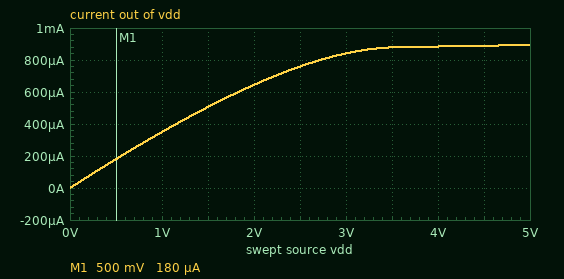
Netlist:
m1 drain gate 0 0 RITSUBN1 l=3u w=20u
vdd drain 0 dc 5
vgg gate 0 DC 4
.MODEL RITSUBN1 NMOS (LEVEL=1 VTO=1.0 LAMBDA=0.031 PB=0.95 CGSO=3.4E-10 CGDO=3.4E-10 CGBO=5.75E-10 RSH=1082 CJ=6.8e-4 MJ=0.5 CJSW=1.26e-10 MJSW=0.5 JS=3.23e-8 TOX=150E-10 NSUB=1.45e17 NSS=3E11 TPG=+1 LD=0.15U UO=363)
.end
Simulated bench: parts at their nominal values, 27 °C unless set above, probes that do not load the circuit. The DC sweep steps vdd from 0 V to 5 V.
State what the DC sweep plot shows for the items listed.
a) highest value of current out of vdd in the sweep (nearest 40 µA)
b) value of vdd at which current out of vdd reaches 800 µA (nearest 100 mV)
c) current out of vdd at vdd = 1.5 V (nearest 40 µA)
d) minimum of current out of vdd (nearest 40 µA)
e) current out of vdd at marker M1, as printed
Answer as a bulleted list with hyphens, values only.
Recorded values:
- 880 µA
- 2.7 V
- 520 µA
- 0 A
- 180 µA
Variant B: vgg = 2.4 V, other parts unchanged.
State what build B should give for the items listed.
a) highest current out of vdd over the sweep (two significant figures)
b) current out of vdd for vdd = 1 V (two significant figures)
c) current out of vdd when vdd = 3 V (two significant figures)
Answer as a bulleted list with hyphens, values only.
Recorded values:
- 300 µA
- 240 µA
- 290 µA
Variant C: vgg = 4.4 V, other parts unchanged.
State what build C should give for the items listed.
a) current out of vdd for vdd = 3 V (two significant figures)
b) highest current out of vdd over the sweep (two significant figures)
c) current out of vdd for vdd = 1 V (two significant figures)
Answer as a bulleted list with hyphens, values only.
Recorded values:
- 930 µA
- 1.1 mA
- 360 µA
